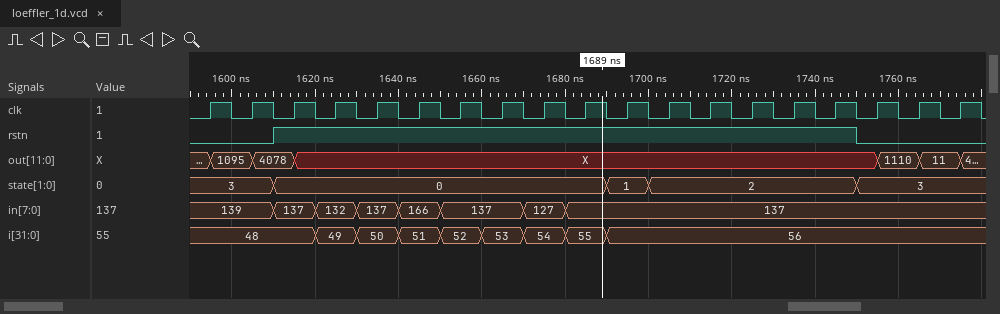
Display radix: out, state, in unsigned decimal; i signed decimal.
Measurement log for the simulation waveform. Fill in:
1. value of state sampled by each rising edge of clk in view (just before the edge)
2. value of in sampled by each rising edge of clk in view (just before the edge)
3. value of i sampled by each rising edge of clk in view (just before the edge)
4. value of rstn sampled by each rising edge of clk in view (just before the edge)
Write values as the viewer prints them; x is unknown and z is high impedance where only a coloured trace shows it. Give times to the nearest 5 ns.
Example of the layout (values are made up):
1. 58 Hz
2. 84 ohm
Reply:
1. 3, 3, 0, 0, 0, 0, 0, 0, 0, 0, 1, 2, 2, 2, 2, 2, 3, 3, 3
2. 139, 139, 137, 132, 137, 166, 137, 137, 127, 137, 137, 137, 137, 137, 137, 137, 137, 137, 137
3. 48, 48, 48, 49, 50, 51, 52, 53, 54, 55, 56, 56, 56, 56, 56, 56, 56, 56, 56
4. 0 0 1 1 1 1 1 1 1 1 1 1 1 1 1 1 0 0 0
